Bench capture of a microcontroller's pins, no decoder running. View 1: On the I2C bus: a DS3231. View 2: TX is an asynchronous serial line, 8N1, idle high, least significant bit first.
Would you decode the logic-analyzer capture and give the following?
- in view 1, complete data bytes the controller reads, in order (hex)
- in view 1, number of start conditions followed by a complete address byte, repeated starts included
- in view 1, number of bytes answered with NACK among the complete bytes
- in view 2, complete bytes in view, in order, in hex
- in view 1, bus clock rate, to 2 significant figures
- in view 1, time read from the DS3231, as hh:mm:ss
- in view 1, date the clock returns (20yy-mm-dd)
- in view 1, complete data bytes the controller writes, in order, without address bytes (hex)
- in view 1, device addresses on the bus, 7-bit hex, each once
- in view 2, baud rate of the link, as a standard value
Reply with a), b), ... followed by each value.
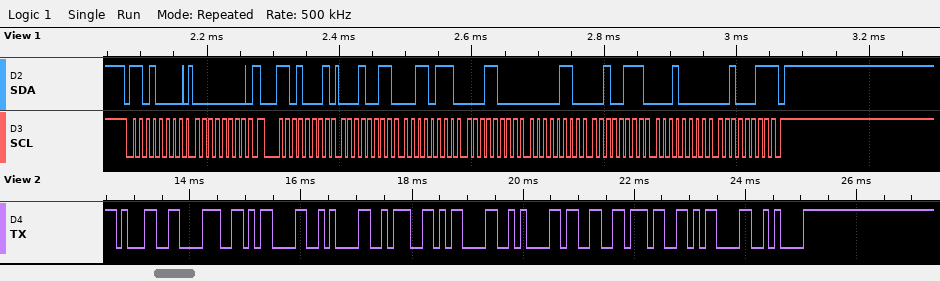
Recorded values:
a) 13 37 18 06 27 10 23
b) 2
c) 1
d) 31 38 0D 0A 3A 0D 0A 33 37 0D 0A
e) 100 kHz
f) 18:37:13
g) 2023-10-27
h) 00
i) 0x68
j) 9600 baud
